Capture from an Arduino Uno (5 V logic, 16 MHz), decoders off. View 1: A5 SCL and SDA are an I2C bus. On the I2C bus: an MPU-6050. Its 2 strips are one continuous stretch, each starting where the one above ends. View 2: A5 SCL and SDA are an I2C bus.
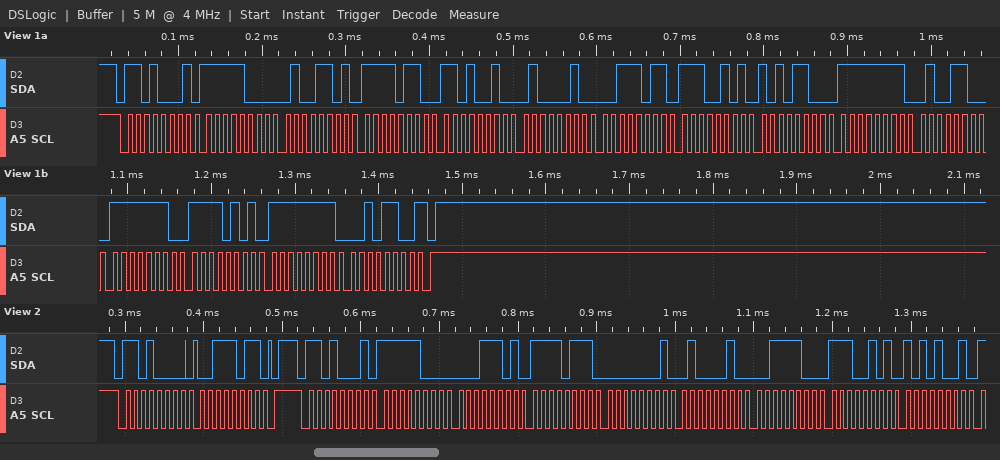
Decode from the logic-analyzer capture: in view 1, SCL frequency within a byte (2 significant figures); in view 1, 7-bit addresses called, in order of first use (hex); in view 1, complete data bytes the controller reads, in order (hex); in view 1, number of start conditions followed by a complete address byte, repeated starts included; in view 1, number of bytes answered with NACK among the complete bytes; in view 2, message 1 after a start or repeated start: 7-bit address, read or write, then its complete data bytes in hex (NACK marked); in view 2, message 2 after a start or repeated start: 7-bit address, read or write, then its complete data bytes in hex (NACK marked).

100 kHz
0x68
F8 4D F6 D2 42 3B E5 AC FF 4C FE F5 FF 2C
1
1
0x68 write: 3B
0x68 read: F8 1D F7 01 42 3C E5 A9
